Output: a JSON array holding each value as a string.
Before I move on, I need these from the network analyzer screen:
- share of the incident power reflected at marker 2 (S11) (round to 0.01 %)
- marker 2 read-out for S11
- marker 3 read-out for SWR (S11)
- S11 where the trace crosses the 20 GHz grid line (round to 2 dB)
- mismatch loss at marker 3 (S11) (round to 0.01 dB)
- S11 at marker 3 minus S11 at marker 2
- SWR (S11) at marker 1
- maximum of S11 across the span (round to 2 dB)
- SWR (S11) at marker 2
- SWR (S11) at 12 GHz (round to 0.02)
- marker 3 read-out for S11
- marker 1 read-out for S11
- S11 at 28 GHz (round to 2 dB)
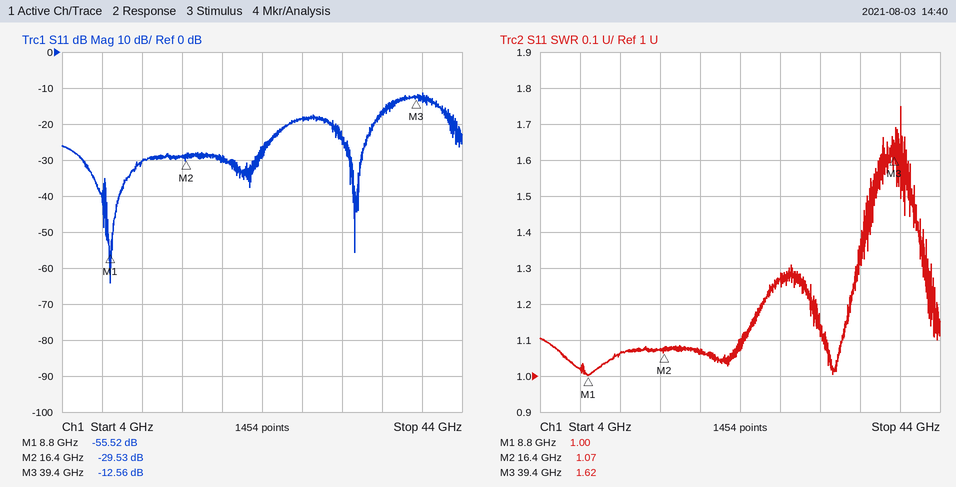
["0.11 %", "-29.53 dB", "1.62", "-30 dB", "0.25 dB", "16.97 dB", "1.00", "-12 dB", "1.07", "1.06", "-12.56 dB", "-55.52 dB", "-18 dB"]
